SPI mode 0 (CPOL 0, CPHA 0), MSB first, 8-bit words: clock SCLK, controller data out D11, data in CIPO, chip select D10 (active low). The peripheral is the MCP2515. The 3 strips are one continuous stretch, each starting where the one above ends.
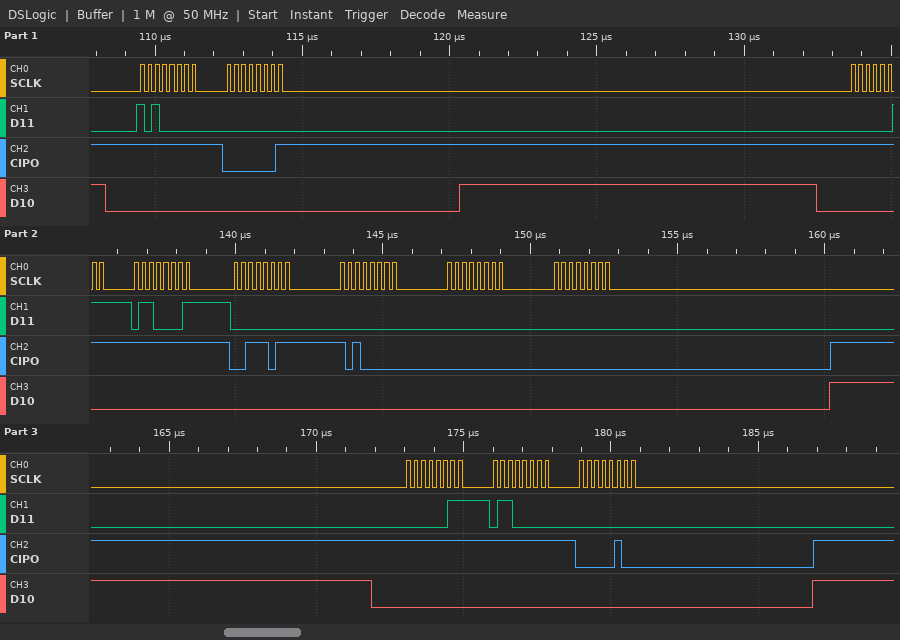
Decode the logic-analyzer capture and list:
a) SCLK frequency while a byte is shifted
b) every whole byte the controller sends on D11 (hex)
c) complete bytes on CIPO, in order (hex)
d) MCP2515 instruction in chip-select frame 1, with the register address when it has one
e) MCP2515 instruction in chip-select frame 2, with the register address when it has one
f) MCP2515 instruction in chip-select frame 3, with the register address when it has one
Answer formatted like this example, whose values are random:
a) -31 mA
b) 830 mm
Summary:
a) 4 MHz
b) A0 00 03 61 00 00 00 00 03 60 00
c) FF 01 FF FF 3B A0 00 00 FF FF 04
d) READ STATUS
e) READ 0x61
f) READ 0x60
